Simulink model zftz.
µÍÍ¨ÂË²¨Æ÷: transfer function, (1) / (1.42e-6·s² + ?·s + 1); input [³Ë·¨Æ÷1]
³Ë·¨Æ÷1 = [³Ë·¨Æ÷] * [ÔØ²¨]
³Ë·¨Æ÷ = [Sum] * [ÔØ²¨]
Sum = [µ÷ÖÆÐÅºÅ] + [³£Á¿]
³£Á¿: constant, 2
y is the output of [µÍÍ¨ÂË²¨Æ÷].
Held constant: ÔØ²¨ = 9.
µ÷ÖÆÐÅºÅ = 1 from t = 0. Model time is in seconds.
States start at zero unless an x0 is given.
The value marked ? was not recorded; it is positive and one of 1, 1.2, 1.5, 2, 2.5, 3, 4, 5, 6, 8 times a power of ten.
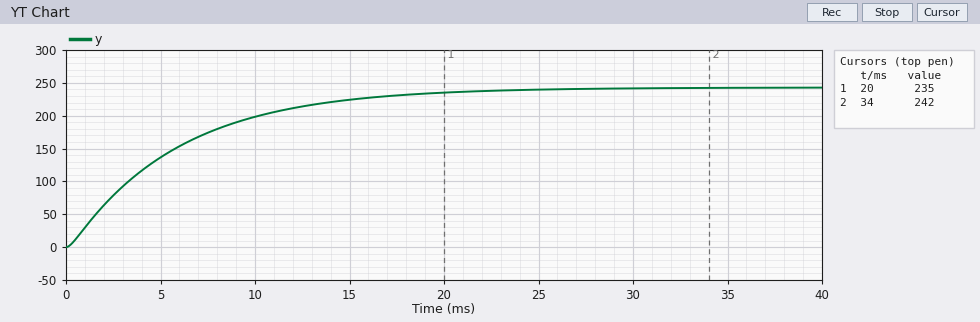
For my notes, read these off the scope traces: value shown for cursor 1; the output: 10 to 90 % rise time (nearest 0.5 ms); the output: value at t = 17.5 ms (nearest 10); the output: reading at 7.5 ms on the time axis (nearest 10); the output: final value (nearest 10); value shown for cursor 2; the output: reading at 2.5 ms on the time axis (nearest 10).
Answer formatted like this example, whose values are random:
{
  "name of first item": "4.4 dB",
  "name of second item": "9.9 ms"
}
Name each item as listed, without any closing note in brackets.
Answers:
{
  "value shown for cursor 1": "235",
  "the output: 10 to 90 % rise time": "12.5 ms",
  "the output: value at t = 17.5 ms": "230",
  "the output: reading at 7.5 ms on the time axis": "170",
  "the output: final value": "240",
  "value shown for cursor 2": "242",
  "the output: reading at 2.5 ms on the time axis": "80"
}
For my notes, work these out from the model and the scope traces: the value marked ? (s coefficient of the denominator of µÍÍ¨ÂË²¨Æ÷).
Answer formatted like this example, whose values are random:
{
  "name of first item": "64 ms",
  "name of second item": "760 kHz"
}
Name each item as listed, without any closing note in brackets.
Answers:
{
  "the value marked ?": "0.006"
}
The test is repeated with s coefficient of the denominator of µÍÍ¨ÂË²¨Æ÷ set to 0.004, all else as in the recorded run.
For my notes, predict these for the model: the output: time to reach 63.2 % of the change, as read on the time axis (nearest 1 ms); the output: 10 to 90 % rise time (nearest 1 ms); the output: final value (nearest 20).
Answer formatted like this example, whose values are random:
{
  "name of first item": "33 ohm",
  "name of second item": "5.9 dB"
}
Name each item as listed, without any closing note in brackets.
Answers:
{
  "the output: time to reach 63.2 % of the change, as read on the time axis": "4 ms",
  "the output: 10 to 90 % rise time": "8 ms",
  "the output: final value": "240"
}
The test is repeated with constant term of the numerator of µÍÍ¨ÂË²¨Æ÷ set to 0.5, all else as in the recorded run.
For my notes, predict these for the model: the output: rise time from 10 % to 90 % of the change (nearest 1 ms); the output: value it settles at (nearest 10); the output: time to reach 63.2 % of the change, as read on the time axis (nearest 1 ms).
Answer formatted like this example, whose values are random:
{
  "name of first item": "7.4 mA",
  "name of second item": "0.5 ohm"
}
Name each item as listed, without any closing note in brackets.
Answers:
{
  "the output: rise time from 10 % to 90 % of the change": "13 ms",
  "the output: value it settles at": "120",
  "the output: time to reach 63.2 % of the change, as read on the time axis": "6 ms"
}
